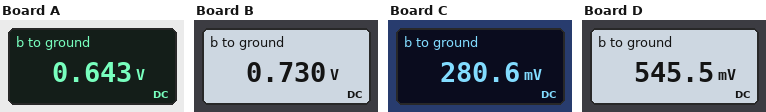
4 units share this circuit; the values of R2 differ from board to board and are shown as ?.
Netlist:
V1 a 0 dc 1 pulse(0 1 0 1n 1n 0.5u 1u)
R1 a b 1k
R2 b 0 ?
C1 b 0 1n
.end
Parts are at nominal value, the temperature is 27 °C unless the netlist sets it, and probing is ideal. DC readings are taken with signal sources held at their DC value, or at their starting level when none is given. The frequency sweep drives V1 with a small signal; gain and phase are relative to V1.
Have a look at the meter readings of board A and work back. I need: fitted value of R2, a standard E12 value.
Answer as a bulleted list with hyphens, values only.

- 1.8 kΩ
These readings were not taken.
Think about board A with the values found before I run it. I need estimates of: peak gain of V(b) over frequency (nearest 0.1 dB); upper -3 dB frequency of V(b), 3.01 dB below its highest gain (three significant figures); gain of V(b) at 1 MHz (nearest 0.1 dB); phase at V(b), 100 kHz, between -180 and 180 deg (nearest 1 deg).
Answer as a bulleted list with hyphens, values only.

- -3.8 dB
- 248 kHz
- -16.2 dB
- -22 deg
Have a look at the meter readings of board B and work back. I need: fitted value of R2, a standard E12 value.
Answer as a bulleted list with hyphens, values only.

- 2.7 kΩ
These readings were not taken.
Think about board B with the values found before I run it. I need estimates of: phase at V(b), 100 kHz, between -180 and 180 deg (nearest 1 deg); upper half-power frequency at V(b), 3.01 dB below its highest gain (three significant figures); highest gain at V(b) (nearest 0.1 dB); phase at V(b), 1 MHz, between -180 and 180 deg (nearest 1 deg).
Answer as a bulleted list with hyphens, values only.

- -25 deg
- 218 kHz
- -2.7 dB
- -78 deg
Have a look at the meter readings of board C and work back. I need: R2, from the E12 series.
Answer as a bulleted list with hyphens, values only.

- 390 Ω
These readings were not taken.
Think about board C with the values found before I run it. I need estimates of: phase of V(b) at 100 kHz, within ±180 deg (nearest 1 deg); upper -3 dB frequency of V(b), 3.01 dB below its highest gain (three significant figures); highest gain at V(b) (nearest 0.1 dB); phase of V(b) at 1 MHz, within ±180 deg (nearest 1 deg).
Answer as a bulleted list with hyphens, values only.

- -10 deg
- 567 kHz
- -11.0 dB
- -60 deg
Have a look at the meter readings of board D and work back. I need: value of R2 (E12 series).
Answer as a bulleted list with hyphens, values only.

- 1.2 kΩ
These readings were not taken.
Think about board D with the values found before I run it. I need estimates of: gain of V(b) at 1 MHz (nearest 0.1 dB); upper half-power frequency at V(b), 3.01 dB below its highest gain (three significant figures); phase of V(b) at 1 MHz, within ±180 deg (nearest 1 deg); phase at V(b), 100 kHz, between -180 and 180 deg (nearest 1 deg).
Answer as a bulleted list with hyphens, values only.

- -16.3 dB
- 292 kHz
- -74 deg
- -19 deg
